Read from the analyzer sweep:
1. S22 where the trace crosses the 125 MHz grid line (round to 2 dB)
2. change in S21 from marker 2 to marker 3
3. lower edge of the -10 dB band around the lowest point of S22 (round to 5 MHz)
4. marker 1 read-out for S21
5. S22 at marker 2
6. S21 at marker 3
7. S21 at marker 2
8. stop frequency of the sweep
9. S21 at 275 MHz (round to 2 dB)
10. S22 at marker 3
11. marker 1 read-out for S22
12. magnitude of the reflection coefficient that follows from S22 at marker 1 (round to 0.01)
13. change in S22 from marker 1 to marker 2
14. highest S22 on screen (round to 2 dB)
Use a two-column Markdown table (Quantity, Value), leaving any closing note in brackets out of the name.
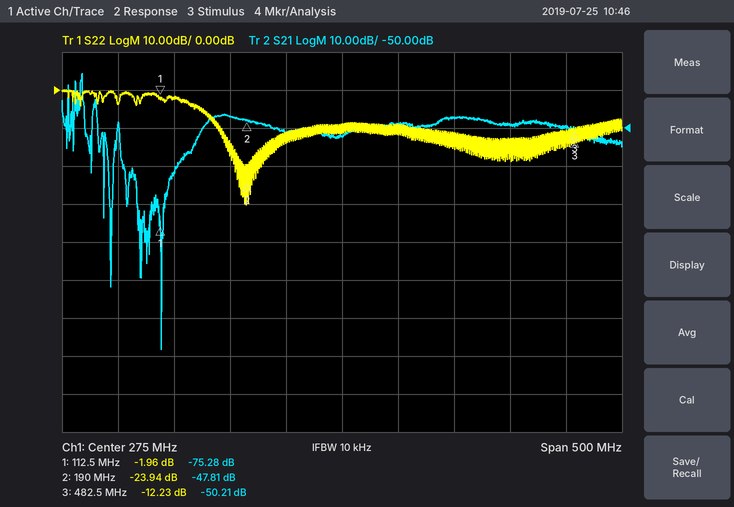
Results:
| Quantity | Value |
|---|---|
| S22 where the trace crosses the 125 MHz grid line | -2 dB |
| change in S21 from marker 2 to marker 3 | -2.40 dB |
| lower edge of the -10 dB band around the lowest point of S22 | 165 MHz |
| marker 1 read-out for S21 | -75.28 dB |
| S22 at marker 2 | -23.94 dB |
| S21 at marker 3 | -50.21 dB |
| S21 at marker 2 | -47.81 dB |
| stop frequency of the sweep | 525 MHz |
| S21 at 275 MHz | -52 dB |
| S22 at marker 3 | -12.23 dB |
| marker 1 read-out for S22 | -1.96 dB |
| magnitude of the reflection coefficient that follows from S22 at marker 1 | 0.80 |
| change in S22 from marker 1 to marker 2 | -21.98 dB |
| highest S22 on screen | 0 dB |
